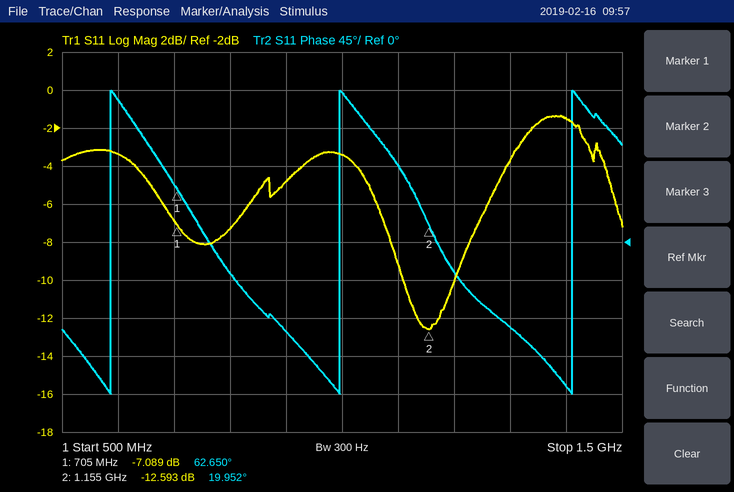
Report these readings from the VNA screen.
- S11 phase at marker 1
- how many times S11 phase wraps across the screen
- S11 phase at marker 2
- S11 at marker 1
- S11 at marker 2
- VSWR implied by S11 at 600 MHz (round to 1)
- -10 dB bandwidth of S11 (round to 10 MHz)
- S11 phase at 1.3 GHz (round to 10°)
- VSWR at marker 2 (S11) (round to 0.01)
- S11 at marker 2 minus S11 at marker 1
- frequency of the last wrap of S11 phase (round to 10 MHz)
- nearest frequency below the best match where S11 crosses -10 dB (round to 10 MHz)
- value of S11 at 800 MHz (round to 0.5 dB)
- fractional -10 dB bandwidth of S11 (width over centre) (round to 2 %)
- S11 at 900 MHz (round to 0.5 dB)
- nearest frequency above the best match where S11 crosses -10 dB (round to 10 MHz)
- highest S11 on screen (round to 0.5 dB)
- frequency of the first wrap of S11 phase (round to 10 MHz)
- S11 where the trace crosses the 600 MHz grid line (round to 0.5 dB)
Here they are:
62.650°
3
19.952°
-7.089 dB
-12.593 dB
5
90 MHz
-100°
1.61
-5.504 dB
1.41 GHz
1.11 GHz
-7.5 dB
8 %
-5.0 dB
1.20 GHz
-1.5 dB
590 MHz
-3.5 dB
